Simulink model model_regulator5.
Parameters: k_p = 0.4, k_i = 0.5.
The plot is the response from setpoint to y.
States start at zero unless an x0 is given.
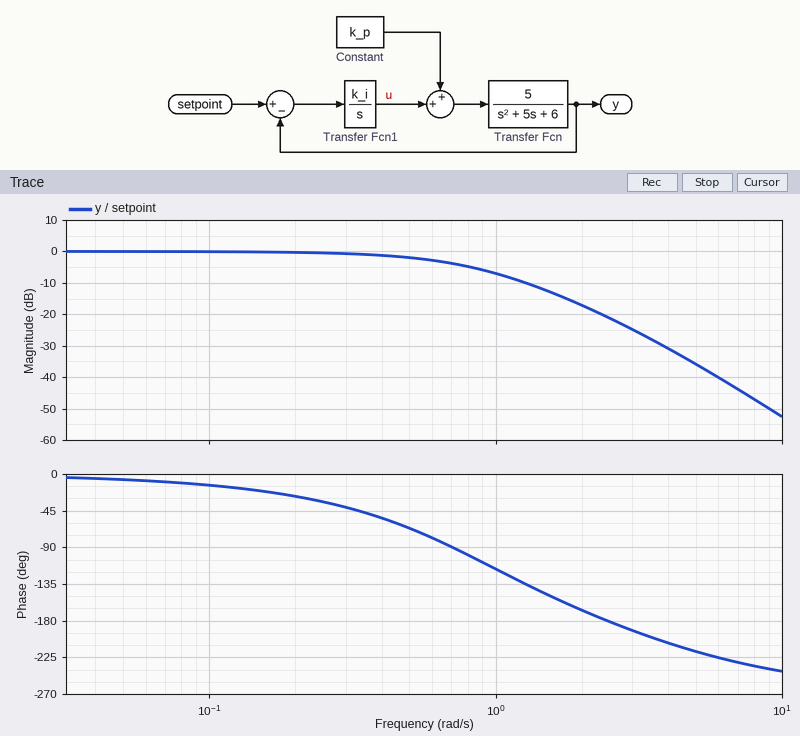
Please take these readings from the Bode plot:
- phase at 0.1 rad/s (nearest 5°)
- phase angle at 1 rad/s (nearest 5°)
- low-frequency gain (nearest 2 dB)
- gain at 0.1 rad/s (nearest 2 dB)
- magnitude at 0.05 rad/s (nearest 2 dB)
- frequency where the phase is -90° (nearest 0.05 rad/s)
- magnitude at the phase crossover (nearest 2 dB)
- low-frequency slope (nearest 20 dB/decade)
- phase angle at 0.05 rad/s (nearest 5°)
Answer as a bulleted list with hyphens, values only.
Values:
- -15°
- -115°
- 0 dB
- 0 dB
- 0 dB
- 0.70 rad/s
- -20 dB
- 0 dB/decade
- -5°
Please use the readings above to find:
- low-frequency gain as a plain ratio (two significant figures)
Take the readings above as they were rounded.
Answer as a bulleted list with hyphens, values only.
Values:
- 1.0
